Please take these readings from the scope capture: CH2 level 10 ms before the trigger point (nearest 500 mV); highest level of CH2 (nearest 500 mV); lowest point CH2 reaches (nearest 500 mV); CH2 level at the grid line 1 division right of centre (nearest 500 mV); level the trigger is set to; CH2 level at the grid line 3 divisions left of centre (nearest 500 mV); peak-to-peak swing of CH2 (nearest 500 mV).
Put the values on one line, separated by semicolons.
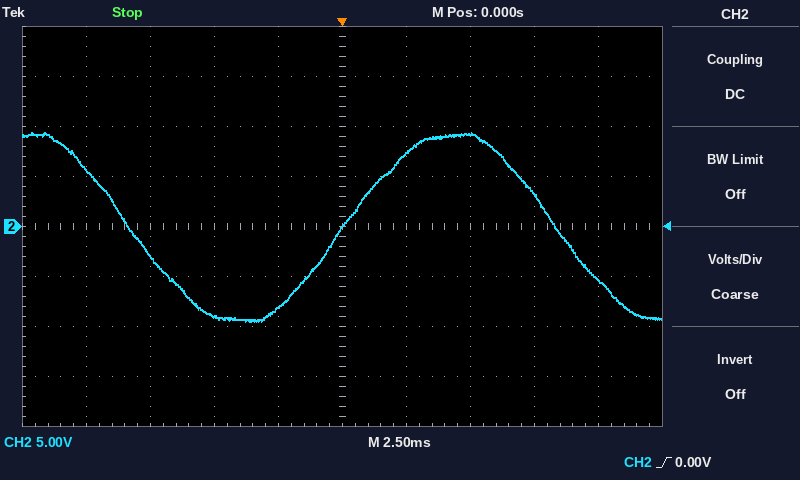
5.5 V; 9.5 V; -9.5 V; 7.5 V; 0.00 V; -3.0 V; 19.0 V
